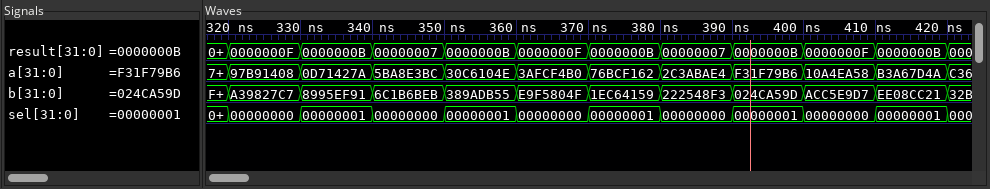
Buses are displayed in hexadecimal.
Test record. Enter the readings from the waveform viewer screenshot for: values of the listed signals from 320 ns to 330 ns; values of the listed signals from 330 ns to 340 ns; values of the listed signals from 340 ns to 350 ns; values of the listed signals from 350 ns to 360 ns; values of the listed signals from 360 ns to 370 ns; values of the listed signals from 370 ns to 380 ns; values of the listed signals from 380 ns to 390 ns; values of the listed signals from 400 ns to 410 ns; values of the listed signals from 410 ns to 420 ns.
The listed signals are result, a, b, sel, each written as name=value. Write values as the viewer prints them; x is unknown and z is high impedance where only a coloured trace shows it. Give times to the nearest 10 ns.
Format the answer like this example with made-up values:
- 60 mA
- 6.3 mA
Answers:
- result=0000000F, a=97B91408, b=A39827C7, sel=00000000
- result=0000000B, a=0D71427A, b=8995EF91, sel=00000001
- result=00000007, a=5BA8E3BC, b=6C1B6BEB, sel=00000000
- result=0000000B, a=30C6104E, b=389ADB55, sel=00000001
- result=0000000F, a=3AFCF4B0, b=E9F5804F, sel=00000000
- result=0000000B, a=76BCF162, b=1EC64159, sel=00000001
- result=00000007, a=2C3ABAE4, b=222548F3, sel=00000000
- result=0000000F, a=10A4EA58, b=ACC5E9D7, sel=00000000
- result=0000000B, a=B3A67D4A, b=EE08CC21, sel=00000001
